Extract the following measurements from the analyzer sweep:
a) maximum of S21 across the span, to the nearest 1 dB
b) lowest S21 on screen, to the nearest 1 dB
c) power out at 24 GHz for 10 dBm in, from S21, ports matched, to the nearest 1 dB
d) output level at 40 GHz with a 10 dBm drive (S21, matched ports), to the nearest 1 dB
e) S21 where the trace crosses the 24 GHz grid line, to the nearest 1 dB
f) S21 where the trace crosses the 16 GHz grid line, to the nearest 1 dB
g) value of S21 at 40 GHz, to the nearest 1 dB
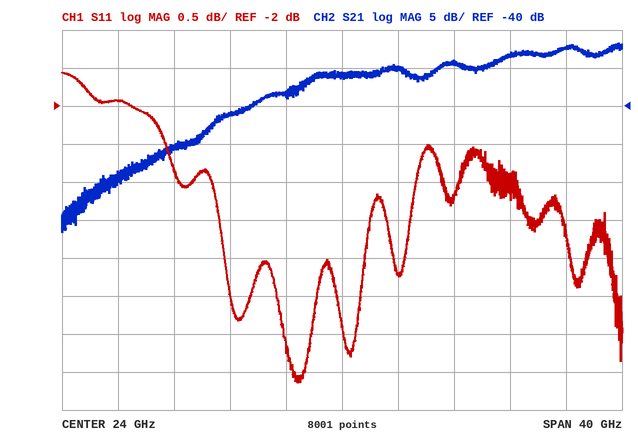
-32 dB
-57 dB
-26 dBm
-22 dBm
-36 dB
-41 dB
-32 dB
